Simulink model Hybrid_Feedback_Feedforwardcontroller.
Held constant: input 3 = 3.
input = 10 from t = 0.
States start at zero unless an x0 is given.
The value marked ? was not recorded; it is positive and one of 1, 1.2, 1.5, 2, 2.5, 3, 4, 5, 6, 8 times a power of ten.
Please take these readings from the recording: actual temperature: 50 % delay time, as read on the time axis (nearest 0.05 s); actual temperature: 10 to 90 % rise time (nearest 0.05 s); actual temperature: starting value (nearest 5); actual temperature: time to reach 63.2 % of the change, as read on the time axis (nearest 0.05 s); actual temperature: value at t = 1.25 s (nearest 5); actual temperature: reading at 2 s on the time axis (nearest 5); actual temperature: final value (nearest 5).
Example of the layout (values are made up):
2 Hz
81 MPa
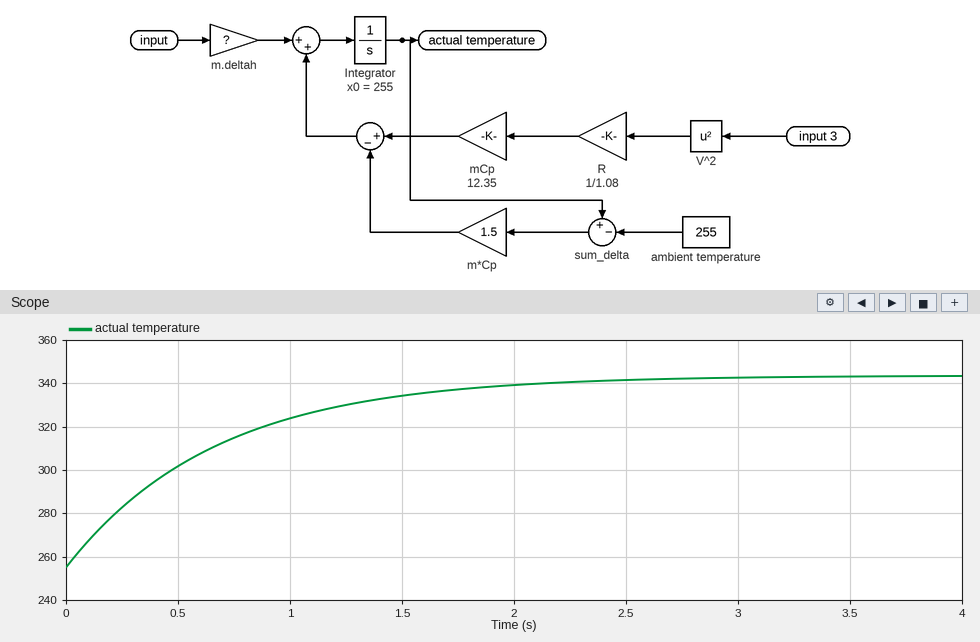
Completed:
0.45 s
1.45 s
255
0.65 s
330
340
345
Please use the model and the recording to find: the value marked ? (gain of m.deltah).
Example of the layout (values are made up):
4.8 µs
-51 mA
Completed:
3
